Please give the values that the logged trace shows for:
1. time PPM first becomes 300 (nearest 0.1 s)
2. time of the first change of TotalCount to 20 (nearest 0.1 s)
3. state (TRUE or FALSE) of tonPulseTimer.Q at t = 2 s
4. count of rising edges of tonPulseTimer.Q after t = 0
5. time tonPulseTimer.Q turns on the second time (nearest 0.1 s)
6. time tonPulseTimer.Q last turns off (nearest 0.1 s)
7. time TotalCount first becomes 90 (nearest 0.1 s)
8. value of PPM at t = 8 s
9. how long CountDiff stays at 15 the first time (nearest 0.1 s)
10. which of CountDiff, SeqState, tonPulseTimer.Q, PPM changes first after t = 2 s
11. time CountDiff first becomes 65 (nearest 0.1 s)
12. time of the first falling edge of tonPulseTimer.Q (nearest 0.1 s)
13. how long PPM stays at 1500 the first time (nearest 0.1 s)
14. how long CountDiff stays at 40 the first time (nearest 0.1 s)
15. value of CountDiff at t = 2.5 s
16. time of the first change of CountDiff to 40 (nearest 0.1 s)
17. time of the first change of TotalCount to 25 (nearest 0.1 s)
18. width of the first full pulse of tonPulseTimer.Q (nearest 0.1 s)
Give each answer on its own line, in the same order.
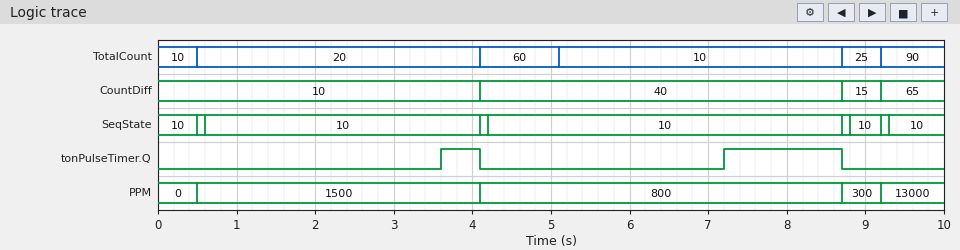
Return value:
8.7 s
0.5 s
FALSE
2
7.2 s
8.7 s
9.2 s
800
0.5 s
tonPulseTimer.Q
9.2 s
4.1 s
3.6 s
4.6 s
10
4.1 s
8.7 s
0.5 s
